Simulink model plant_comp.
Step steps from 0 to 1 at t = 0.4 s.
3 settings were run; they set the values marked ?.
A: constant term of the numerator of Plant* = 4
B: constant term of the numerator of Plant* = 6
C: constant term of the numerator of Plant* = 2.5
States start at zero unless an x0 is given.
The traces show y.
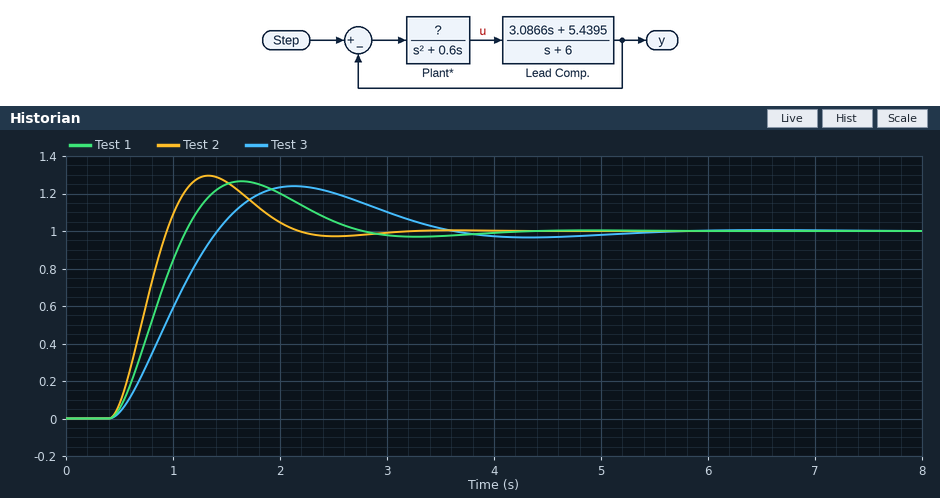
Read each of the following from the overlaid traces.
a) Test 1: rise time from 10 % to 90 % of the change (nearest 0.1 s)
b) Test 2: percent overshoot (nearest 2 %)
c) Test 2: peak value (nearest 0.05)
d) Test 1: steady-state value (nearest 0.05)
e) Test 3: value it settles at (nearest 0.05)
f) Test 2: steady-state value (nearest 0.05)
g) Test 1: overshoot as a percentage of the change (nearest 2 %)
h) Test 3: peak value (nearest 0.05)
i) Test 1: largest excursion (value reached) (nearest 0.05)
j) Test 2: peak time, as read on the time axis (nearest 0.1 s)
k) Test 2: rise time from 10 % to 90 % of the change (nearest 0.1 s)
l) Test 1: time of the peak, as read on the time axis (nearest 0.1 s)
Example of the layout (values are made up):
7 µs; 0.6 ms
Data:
0.5 s; 30 %; 1.30; 1.00; 1.00; 1.00; 26 %; 1.25; 1.25; 1.3 s; 0.4 s; 1.6 s
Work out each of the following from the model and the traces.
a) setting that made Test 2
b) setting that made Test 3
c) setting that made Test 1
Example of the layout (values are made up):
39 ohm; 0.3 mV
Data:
B; C; A
